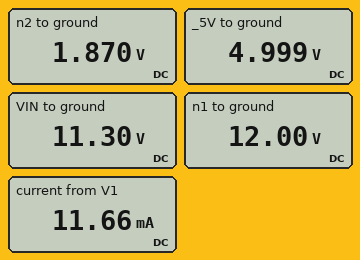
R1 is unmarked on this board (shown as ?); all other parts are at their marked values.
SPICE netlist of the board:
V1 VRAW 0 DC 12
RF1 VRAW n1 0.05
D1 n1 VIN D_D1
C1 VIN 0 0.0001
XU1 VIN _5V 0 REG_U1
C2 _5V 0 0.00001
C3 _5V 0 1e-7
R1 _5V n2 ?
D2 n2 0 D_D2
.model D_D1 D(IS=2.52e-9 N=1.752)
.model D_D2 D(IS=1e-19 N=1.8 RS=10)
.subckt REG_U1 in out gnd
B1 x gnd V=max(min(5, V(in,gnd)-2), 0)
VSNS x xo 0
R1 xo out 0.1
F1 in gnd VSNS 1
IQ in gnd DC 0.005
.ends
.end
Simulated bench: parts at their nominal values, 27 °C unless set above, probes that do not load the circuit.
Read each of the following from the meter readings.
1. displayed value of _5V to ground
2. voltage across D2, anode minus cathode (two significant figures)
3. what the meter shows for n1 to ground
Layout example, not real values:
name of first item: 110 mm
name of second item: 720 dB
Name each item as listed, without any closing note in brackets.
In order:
displayed value of _5V to ground: 4.999 V
voltage across D2, anode minus cathode: 1.9 V
what the meter shows for n1 to ground: 12.00 V
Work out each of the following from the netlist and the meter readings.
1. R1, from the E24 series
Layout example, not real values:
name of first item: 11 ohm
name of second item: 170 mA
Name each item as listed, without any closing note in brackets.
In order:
R1, from the E24 series: 470 Ω
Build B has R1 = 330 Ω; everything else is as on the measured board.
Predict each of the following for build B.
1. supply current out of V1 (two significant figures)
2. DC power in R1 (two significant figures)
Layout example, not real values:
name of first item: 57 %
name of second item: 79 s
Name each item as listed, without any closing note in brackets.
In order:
supply current out of V1: 14 mA
DC power in R1: 29 mW
